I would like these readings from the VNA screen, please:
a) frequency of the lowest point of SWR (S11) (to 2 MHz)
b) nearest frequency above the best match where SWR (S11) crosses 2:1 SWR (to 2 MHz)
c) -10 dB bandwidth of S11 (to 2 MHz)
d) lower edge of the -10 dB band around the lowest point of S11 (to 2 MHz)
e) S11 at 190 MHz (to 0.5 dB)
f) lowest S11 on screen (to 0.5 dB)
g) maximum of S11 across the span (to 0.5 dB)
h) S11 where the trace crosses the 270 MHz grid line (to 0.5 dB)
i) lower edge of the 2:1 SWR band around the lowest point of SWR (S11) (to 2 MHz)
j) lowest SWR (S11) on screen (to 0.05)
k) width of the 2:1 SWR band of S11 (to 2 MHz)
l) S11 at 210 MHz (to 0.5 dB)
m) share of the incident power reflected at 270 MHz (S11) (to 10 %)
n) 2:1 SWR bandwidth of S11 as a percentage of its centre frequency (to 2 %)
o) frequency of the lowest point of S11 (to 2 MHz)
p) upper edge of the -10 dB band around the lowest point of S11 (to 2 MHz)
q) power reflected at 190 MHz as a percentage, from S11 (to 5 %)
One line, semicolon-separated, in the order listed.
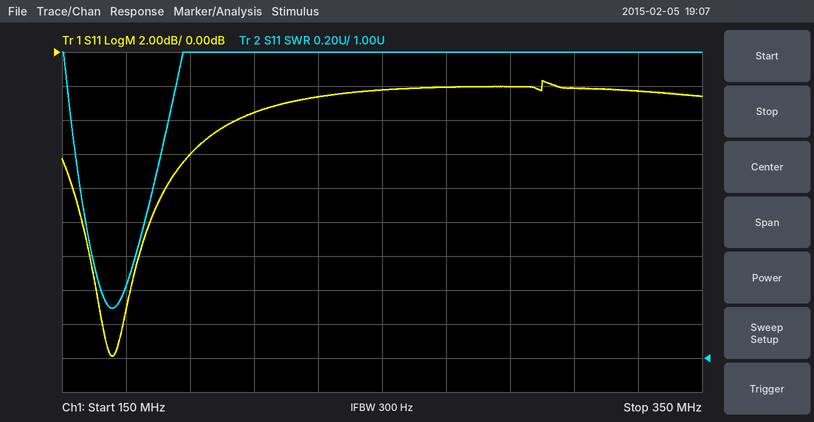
166 MHz; 178 MHz; 22 MHz; 156 MHz; -6.0 dB; -18.0 dB; -1.5 dB; -2.0 dB; 156 MHz; 1.30; 22 MHz; -3.5 dB; 60 %; 14 %; 166 MHz; 178 MHz; 25 %
